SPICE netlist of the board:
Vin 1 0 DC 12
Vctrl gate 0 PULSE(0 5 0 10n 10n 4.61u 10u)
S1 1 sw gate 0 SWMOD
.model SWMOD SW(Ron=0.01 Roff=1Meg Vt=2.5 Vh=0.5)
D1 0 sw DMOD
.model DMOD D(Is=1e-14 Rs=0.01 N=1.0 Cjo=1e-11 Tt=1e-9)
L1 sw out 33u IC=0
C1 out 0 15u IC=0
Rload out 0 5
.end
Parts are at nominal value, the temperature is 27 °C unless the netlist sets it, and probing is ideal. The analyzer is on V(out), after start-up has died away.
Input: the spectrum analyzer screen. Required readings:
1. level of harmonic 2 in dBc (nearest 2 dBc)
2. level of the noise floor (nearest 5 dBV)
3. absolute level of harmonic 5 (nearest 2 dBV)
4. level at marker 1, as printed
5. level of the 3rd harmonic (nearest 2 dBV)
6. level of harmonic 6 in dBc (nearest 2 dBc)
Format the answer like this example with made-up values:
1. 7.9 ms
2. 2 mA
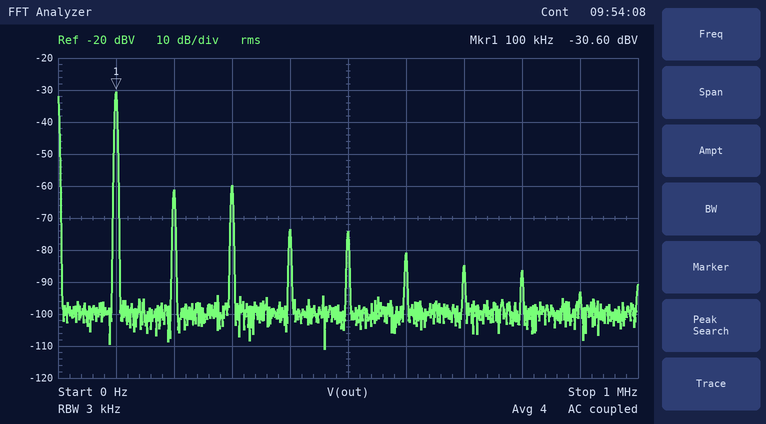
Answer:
1. -30 dBc
2. -100 dBV
3. -74 dBV
4. -30.60 dBV
5. -60 dBV
6. -50 dBc
